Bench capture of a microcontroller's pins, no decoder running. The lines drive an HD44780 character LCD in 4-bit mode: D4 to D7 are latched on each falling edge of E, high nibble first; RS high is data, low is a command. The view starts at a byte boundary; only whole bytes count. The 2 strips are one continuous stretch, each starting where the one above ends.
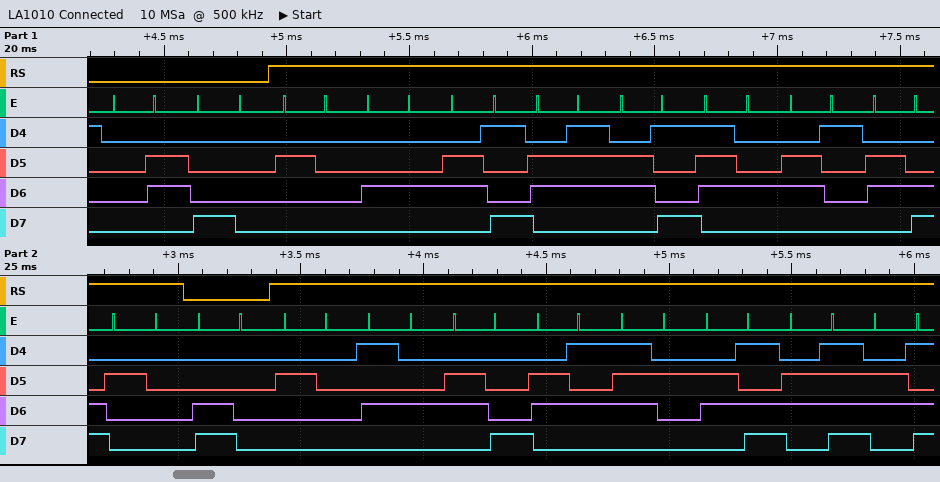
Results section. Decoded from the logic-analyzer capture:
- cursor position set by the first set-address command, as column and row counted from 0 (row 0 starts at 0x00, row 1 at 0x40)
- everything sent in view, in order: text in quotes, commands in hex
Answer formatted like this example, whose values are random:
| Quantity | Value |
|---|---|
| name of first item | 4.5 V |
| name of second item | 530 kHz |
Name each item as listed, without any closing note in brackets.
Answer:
| Quantity | Value |
|---|---|
| cursor position set by the first set-address command, as column and row counted from 0 | column 0, row 0 |
| everything sent in view, in order: text in quotes, commands in hex | 0x06 0x80 " Digital " 0xC0 " Thermom" |
